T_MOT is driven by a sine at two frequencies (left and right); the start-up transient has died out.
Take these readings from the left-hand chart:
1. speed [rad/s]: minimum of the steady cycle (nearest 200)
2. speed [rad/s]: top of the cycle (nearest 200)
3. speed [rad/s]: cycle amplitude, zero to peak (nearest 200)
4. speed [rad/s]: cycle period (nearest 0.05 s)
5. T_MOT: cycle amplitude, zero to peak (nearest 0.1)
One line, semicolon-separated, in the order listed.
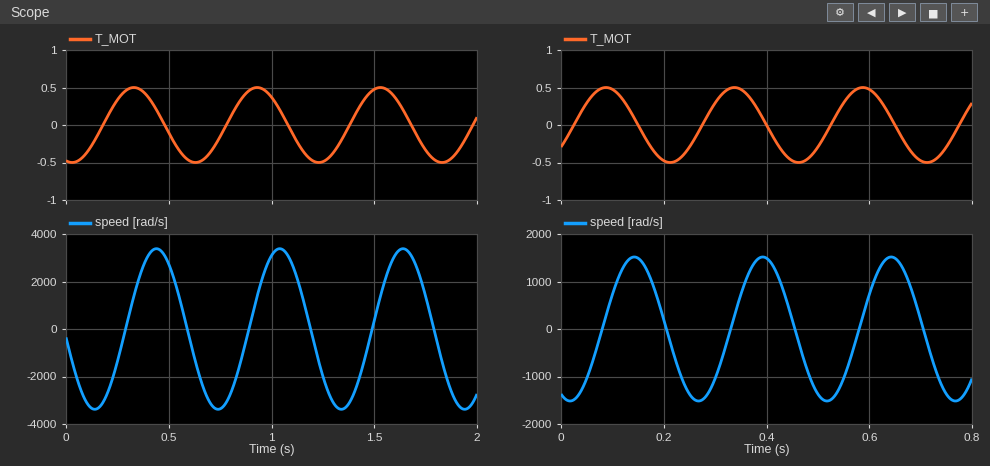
-3400; 3400; 3400; 0.60 s; 0.5
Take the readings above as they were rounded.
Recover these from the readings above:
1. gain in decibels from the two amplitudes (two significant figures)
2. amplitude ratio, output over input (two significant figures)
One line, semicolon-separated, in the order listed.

77 dB; 6800
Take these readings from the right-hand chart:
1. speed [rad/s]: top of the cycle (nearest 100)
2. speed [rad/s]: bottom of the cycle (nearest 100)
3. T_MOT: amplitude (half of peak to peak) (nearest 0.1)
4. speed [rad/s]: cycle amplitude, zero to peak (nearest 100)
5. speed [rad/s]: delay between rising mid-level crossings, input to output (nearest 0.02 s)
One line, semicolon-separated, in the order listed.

1500; -1500; 0.5; 1500; 0.06 s
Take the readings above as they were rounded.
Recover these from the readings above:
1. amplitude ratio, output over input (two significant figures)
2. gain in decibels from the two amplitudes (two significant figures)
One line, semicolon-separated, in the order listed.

3000; 70 dB
